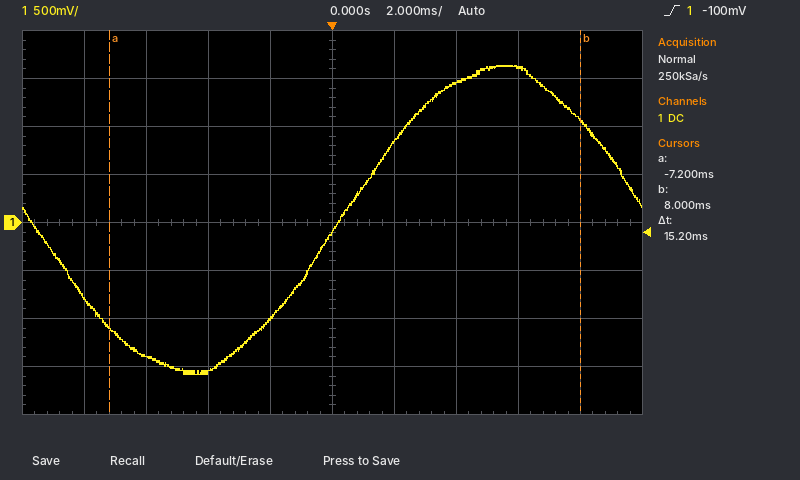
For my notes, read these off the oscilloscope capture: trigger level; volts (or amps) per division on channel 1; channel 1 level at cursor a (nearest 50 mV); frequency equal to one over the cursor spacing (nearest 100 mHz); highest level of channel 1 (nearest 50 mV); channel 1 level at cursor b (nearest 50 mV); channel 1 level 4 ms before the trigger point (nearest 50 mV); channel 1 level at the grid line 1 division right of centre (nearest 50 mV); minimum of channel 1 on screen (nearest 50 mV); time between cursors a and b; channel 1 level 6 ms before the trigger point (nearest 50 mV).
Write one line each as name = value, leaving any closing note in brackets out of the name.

trigger level = -100 mV
volts (or amps) per division on channel 1 = 500 mV
channel 1 level at cursor a = -1.10 V
frequency equal to one over the cursor spacing = 65.8 Hz
highest level of channel 1 = 1.65 V
channel 1 level at cursor b = 1.05 V
channel 1 level 4 ms before the trigger point = -1.55 V
channel 1 level at the grid line 1 division right of centre = 850 mV
minimum of channel 1 on screen = -1.60 V
time between cursors a and b = 15.2 ms
channel 1 level 6 ms before the trigger point = -1.40 V
